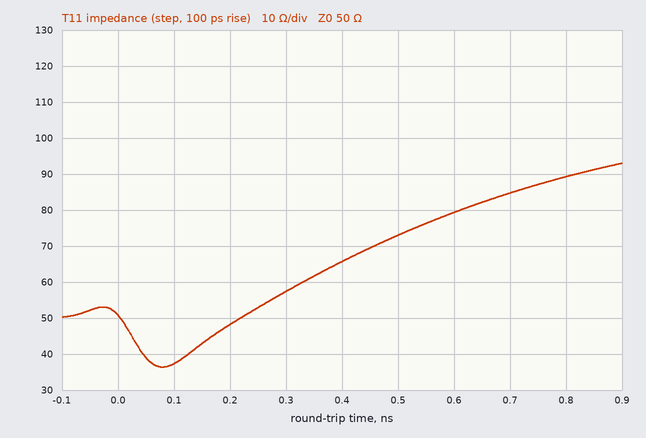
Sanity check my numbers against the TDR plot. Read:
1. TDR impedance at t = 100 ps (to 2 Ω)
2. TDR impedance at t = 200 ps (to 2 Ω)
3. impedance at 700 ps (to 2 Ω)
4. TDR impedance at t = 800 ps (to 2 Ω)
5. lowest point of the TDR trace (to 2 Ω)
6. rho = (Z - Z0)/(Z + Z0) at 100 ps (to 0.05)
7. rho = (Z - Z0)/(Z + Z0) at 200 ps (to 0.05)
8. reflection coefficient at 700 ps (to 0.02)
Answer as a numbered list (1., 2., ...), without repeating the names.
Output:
1. 38 Ω
2. 48 Ω
3. 84 Ω
4. 90 Ω
5. 36 Ω
6. -0.15
7. 0.00
8. +0.26
